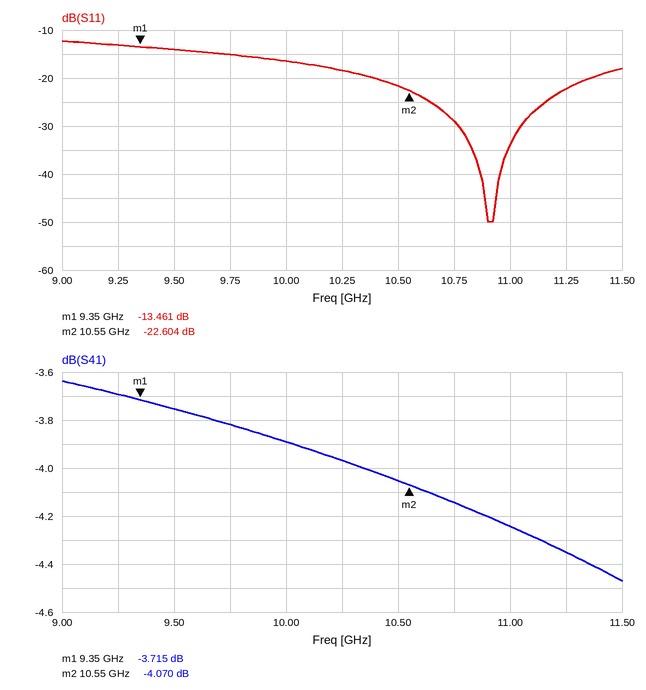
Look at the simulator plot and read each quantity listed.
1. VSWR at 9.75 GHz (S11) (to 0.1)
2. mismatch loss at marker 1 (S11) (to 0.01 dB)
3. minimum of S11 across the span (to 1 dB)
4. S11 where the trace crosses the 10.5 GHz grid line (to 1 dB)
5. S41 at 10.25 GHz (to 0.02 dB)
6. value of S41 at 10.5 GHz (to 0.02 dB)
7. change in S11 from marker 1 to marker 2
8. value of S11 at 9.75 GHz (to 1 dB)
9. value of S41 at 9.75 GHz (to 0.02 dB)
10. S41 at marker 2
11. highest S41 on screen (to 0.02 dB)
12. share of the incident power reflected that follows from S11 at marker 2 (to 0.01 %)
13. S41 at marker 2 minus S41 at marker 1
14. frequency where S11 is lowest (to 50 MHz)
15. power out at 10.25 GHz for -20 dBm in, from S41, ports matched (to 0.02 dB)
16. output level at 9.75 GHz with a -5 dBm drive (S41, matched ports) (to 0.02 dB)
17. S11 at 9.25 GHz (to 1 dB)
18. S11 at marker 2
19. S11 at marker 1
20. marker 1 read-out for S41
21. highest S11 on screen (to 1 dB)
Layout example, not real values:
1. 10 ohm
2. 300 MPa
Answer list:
1. 1.4
2. 0.20 dB
3. -50 dB
4. -22 dB
5. -3.96 dB
6. -4.06 dB
7. -9.143 dB
8. -15 dB
9. -3.82 dB
10. -4.070 dB
11. -3.64 dB
12. 0.55 %
13. -0.355 dB
14. 10.90 GHz
15. -23.96 dBm
16. -8.82 dBm
17. -13 dB
18. -22.604 dB
19. -13.461 dB
20. -3.715 dB
21. -12 dB
